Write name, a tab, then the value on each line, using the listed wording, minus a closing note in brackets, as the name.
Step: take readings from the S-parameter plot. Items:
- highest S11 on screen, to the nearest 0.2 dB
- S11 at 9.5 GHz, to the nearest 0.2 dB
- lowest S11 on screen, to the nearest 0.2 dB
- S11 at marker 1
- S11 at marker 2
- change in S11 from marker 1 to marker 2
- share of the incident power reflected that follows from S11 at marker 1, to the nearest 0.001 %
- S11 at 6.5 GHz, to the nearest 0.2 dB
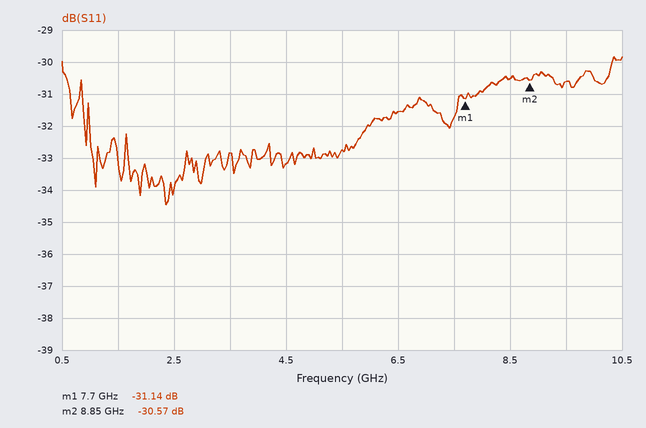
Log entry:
highest S11 on screen, to the nearest 0.2 dB	-29.8 dB
S11 at 9.5 GHz, to the nearest 0.2 dB	-30.6 dB
lowest S11 on screen, to the nearest 0.2 dB	-34.4 dB
S11 at marker 1	-31.14 dB
S11 at marker 2	-30.57 dB
change in S11 from marker 1 to marker 2	0.57 dB
share of the incident power reflected that follows from S11 at marker 1, to the nearest 0.001 %	0.077 %
S11 at 6.5 GHz, to the nearest 0.2 dB	-31.6 dB
